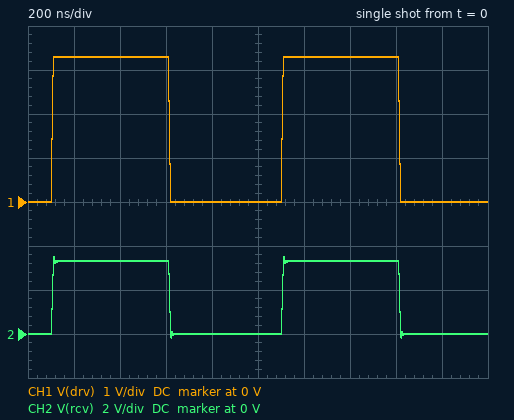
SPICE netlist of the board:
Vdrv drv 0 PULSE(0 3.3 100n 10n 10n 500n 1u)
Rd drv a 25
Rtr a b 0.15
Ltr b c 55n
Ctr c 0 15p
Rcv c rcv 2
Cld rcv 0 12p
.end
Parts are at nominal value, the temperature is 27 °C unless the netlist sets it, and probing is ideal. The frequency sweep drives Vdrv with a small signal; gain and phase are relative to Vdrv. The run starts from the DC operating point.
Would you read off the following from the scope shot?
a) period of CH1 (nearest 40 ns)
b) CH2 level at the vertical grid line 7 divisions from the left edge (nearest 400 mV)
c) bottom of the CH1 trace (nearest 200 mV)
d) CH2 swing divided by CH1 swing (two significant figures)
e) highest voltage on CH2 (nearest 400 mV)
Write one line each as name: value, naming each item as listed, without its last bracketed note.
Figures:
period of CH1: 1.00 µs
CH2 level at the vertical grid line 7 divisions from the left edge: 3.2 V
bottom of the CH1 trace: 0 V
CH2 swing divided by CH1 swing: 1.1
highest voltage on CH2: 3.6 V
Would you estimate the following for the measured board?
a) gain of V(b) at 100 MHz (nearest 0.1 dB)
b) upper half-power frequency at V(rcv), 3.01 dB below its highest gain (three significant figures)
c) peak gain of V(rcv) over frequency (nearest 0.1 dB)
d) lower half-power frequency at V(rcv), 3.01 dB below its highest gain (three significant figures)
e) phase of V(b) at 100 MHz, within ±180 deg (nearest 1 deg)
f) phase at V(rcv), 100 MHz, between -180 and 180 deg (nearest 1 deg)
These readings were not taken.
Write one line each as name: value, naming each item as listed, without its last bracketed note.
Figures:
gain of V(b) at 100 MHz: -3.2 dB
upper half-power frequency at V(rcv), 3.01 dB below its highest gain: 154 MHz
peak gain of V(rcv) over frequency: 5.3 dB
lower half-power frequency at V(rcv), 3.01 dB below its highest gain: 71.2 MHz
phase of V(b) at 100 MHz, within ±180 deg: -45 deg
phase at V(rcv), 100 MHz, between -180 and 180 deg: -47 deg
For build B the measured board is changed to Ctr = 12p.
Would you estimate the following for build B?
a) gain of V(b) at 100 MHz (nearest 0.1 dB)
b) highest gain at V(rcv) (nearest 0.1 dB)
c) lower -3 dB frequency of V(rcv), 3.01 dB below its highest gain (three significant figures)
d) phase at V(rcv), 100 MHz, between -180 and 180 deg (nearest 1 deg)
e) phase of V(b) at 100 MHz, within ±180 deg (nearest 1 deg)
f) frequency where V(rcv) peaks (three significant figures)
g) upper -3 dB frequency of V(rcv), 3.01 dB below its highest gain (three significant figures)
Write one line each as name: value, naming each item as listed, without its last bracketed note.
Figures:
gain of V(b) at 100 MHz: -2.2 dB
highest gain at V(rcv): 5.7 dB
lower -3 dB frequency of V(rcv), 3.01 dB below its highest gain: 80.8 MHz
phase at V(rcv), 100 MHz, between -180 and 180 deg: -39 deg
phase of V(b) at 100 MHz, within ±180 deg: -38 deg
frequency where V(rcv) peaks: 128 MHz
upper -3 dB frequency of V(rcv), 3.01 dB below its highest gain: 162 MHz
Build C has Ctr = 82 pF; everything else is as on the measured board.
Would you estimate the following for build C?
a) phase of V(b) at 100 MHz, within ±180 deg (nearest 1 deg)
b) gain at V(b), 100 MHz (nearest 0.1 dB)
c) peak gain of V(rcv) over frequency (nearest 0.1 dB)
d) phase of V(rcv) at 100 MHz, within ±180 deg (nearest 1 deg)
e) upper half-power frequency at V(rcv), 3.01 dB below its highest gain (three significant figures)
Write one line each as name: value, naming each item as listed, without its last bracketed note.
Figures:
phase of V(b) at 100 MHz, within ±180 deg: 55 deg
gain at V(b), 100 MHz: -4.8 dB
peak gain of V(rcv) over frequency: 1.0 dB
phase of V(rcv) at 100 MHz, within ±180 deg: -126 deg
upper half-power frequency at V(rcv), 3.01 dB below its highest gain: 81.2 MHz
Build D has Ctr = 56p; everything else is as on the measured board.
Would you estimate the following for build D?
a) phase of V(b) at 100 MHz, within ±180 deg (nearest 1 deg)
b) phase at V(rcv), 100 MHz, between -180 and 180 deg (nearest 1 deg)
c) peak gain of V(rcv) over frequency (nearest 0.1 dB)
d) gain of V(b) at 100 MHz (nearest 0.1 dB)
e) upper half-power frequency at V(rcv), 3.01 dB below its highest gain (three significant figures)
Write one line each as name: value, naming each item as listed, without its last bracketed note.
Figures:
phase of V(b) at 100 MHz, within ±180 deg: 66 deg
phase at V(rcv), 100 MHz, between -180 and 180 deg: -115 deg
peak gain of V(rcv) over frequency: 2.0 dB
gain of V(b) at 100 MHz: -7.9 dB
upper half-power frequency at V(rcv), 3.01 dB below its highest gain: 97.4 MHz
